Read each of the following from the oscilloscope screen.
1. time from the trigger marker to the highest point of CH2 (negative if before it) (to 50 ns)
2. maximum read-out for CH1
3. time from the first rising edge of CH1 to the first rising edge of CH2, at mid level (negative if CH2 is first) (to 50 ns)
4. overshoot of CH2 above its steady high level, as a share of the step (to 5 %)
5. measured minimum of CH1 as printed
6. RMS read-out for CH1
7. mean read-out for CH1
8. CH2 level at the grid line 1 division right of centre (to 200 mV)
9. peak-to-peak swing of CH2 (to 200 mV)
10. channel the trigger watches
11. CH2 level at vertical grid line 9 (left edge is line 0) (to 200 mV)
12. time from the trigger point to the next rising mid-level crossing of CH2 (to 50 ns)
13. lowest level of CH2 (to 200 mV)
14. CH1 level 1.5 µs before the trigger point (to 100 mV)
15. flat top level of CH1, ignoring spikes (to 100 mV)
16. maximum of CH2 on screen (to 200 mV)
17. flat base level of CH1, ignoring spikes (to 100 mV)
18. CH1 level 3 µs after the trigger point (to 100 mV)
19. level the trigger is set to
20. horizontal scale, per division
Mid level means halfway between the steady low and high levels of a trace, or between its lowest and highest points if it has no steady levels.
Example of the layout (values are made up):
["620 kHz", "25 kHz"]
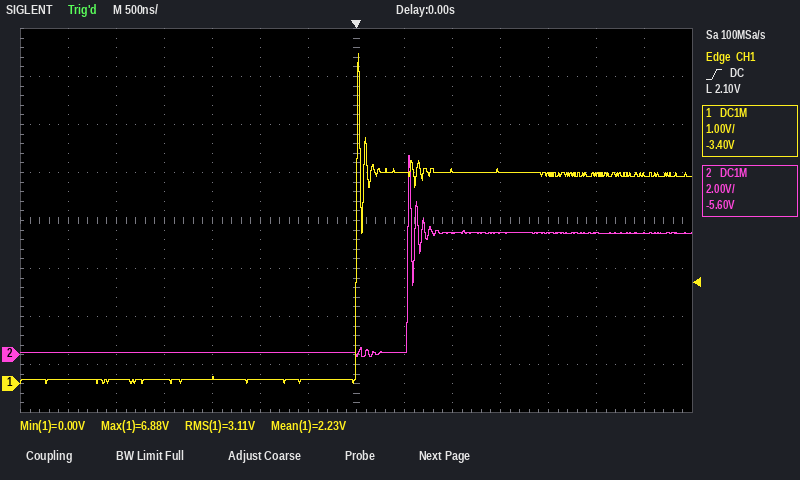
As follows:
["+550 ns", "6.88 V", "+550 ns", "65 %", "0.00 V", "3.11 V", "2.23 V", "0.0 V", "8.4 V", "CH1", "5.0 V", "550 ns", "0.0 V", "100 mV", "4.4 V", "8.4 V", "100 mV", "4.4 V", "2.10 V", "500 ns"]
